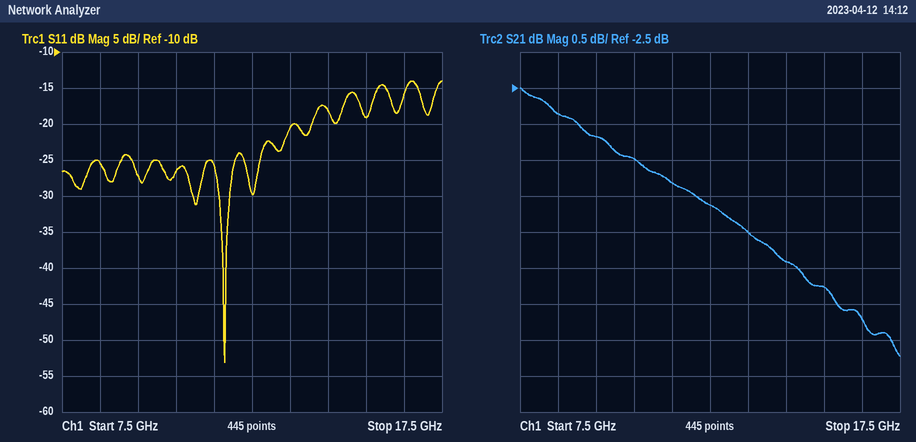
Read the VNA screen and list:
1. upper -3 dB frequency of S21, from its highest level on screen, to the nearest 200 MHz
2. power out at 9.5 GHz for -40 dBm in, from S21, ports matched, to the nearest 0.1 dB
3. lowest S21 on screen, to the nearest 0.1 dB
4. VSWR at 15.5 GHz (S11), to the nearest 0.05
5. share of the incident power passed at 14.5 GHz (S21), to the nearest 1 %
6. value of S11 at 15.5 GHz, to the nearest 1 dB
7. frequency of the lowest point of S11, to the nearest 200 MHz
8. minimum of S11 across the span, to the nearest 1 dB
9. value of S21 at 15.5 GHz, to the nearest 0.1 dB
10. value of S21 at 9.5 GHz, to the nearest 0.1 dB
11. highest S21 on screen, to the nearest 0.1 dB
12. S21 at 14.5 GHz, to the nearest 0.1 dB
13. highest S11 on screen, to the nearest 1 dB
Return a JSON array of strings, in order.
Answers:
["15.8 GHz", "-43.2 dBm", "-6.2 dB", "1.25", "32 %", "-19 dB", "11.8 GHz", "-53 dB", "-5.3 dB", "-3.2 dB", "-2.5 dB", "-4.9 dB", "-14 dB"]
